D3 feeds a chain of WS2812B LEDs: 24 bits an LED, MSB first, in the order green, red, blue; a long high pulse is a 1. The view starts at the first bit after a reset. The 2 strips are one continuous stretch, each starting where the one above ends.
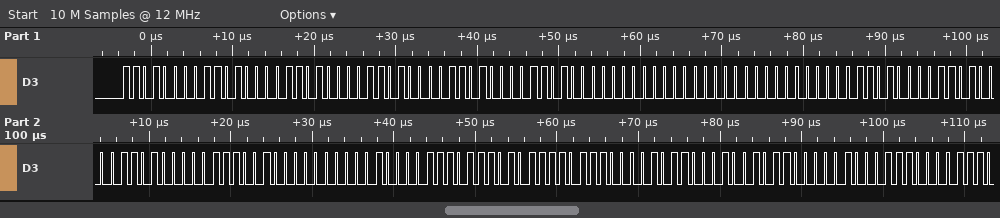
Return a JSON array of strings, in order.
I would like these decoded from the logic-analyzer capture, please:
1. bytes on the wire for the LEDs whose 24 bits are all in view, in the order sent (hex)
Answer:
["D0 D0 D0 D0 D0 D0 00 00 00 D0 D0 D0 72 00 43 BA F7 0B 12 C1 1C"]
